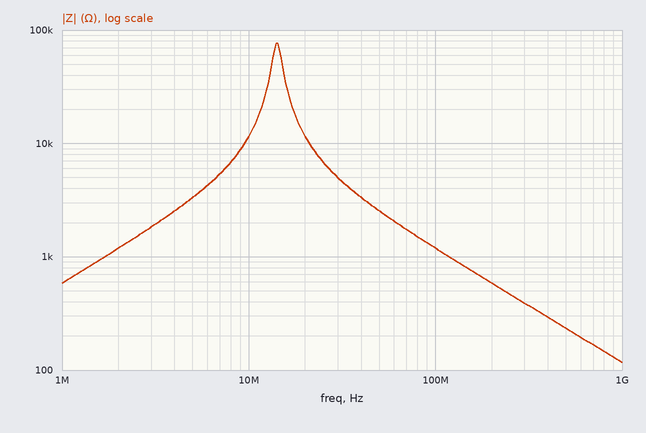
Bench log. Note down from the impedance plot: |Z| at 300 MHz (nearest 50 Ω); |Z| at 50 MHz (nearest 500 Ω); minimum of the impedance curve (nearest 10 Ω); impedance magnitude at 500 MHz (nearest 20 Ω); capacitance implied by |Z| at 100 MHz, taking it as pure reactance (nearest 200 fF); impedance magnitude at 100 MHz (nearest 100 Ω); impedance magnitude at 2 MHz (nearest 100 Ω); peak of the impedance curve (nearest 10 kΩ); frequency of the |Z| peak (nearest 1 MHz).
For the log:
400 Ω
2.5 kΩ
120 Ω
240 Ω
1.4 pF
1.2 kΩ
1.2 kΩ
80 kΩ
14 MHz
